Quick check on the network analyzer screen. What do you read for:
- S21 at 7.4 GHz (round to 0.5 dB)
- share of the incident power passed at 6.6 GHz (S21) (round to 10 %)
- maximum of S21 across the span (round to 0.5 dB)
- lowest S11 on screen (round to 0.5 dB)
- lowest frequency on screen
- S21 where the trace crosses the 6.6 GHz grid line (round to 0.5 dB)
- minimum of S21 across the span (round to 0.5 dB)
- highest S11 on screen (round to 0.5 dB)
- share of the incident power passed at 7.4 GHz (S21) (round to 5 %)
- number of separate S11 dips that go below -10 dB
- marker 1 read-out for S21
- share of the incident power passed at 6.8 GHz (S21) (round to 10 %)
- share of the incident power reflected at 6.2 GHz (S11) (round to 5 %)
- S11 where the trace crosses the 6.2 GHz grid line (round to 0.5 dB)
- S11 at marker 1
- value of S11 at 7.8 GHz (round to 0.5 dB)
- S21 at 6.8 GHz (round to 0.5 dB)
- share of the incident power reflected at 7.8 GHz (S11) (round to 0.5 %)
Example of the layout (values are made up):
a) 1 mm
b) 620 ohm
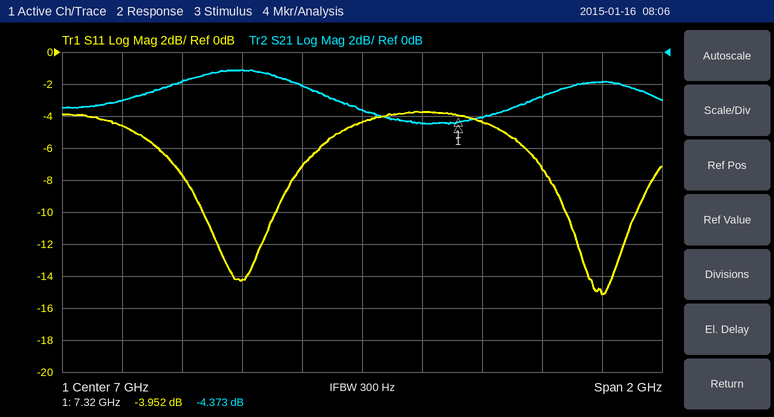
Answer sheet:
a) -4.0 dB
b) 80 %
c) -1.0 dB
d) -15.0 dB
e) 6 GHz
f) -1.0 dB
g) -4.5 dB
h) -3.5 dB
i) 40 %
j) 2
k) -4.373 dB
l) 60 %
m) 35 %
n) -4.5 dB
o) -3.952 dB
p) -15.0 dB
q) -2.0 dB
r) 3.0 %
